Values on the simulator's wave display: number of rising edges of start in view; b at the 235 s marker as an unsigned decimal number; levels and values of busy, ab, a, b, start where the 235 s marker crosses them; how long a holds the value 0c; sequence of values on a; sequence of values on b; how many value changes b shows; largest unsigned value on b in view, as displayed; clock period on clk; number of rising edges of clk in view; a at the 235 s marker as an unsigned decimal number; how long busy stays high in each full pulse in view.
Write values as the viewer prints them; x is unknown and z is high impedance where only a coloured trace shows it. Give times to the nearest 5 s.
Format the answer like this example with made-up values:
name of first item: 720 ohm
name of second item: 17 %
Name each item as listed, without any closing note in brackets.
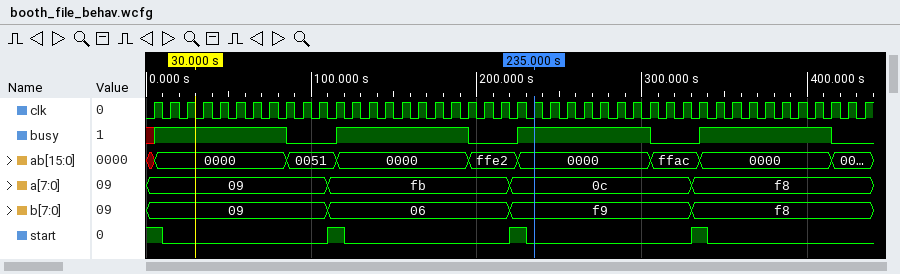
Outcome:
number of rising edges of start in view: 3
b at the 235 s marker as an unsigned decimal number: 249
levels and values of busy, ab, a, b, start where the 235 s marker crosses them: busy=1, ab=0000, a=0c, b=f9, start=0
how long a holds the value 0c: 110 s
sequence of values on a: 09, fb, 0c, f8
sequence of values on b: 09, 06, f9, f8
how many value changes b shows: 3
largest unsigned value on b in view, as displayed: f9
clock period on clk: 10 s
number of rising edges of clk in view: 44
a at the 235 s marker as an unsigned decimal number: 12
how long busy stays high in each full pulse in view: 80 s, 80 s, 80 s
